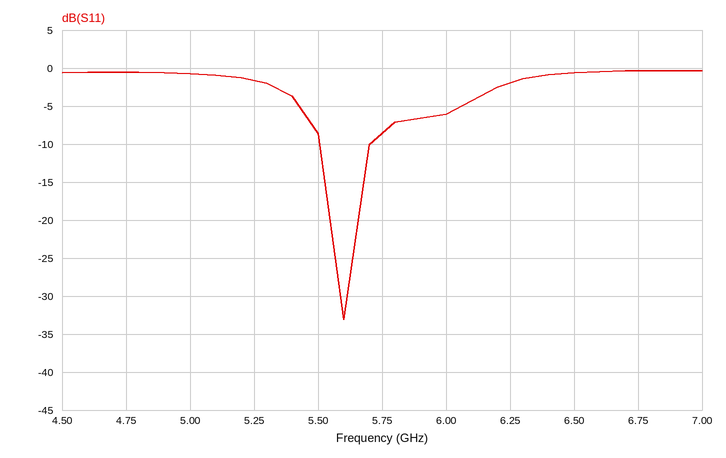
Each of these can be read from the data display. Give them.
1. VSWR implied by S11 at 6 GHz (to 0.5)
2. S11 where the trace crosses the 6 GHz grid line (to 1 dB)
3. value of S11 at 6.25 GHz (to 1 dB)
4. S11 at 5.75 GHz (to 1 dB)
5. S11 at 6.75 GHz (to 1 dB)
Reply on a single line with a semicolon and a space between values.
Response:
3.0; -6 dB; -2 dB; -9 dB; 0 dB
